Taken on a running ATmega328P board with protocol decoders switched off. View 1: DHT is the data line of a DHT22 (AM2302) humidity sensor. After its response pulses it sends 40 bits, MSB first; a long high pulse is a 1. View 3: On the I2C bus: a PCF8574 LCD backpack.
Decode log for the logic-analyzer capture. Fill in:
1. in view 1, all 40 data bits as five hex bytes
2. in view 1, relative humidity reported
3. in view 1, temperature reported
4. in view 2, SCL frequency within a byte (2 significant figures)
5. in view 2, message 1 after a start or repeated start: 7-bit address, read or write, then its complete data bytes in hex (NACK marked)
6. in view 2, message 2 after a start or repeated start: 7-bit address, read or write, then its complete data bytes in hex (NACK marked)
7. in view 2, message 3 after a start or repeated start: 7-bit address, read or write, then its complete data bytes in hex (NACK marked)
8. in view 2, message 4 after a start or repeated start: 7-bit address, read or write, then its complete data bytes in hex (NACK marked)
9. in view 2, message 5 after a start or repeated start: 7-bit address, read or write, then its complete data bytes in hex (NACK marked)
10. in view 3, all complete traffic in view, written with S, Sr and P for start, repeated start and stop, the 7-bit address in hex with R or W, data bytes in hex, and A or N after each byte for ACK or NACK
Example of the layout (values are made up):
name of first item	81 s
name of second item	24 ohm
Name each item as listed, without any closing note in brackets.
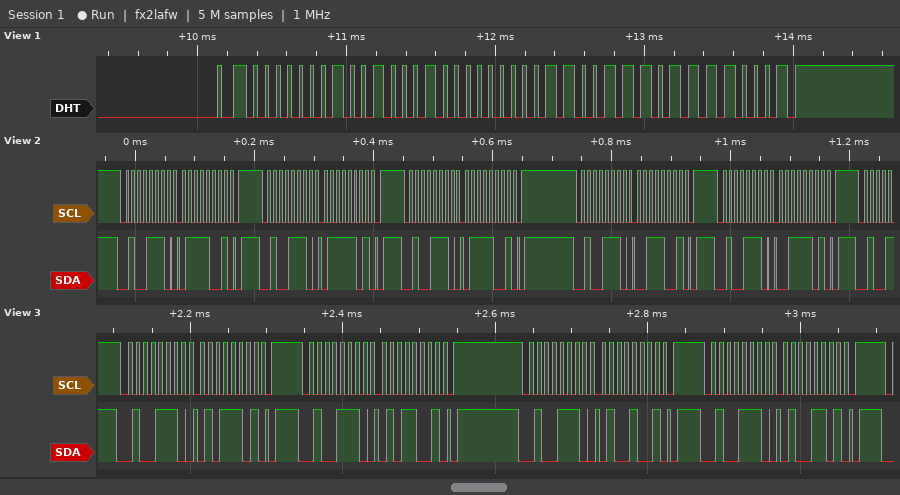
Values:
in view 1, all 40 data bits as five hex bytes	01 22 00 CE F1
in view 1, relative humidity reported	29.0 %
in view 1, temperature reported	20.6 °C
in view 2, SCL frequency within a byte	100 kHz
in view 2, message 1 after a start or repeated start: 7-bit address, read or write, then its complete data bytes in hex	0x27 write: 79
in view 2, message 2 after a start or repeated start: 7-bit address, read or write, then its complete data bytes in hex	0x27 write: 7D
in view 2, message 3 after a start or repeated start: 7-bit address, read or write, then its complete data bytes in hex	0x27 write: 79
in view 2, message 4 after a start or repeated start: 7-bit address, read or write, then its complete data bytes in hex	0x27 write: 39
in view 2, message 5 after a start or repeated start: 7-bit address, read or write, then its complete data bytes in hex	0x27 write: 3D
in view 3, all complete traffic in view, written with S, Sr and P for start, repeated start and stop, the 7-bit address in hex with R or W, data bytes in hex, and A or N after each byte for ACK or NACK	S 27W A 5D A P S 27W A 59 A P S 27W A 49 A P S 27W A 4D A P
